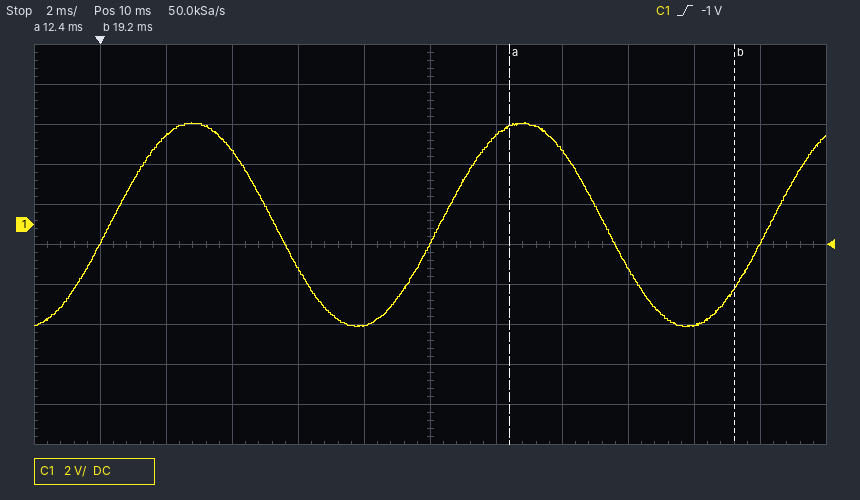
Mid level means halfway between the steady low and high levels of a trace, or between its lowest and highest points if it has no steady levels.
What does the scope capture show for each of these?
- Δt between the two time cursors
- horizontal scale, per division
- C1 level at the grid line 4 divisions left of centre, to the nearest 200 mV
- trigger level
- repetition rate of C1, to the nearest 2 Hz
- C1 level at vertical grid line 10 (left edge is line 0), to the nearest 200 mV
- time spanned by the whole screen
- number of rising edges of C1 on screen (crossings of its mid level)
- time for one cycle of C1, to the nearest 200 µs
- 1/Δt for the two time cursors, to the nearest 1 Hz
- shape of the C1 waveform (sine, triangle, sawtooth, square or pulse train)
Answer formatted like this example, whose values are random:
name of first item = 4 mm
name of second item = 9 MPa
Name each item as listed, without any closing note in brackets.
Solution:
Δt between the two time cursors = 6.8 ms
horizontal scale, per division = 2 ms
C1 level at the grid line 4 divisions left of centre, to the nearest 200 mV = 4.4 V
trigger level = -1 V
repetition rate of C1, to the nearest 2 Hz = 100 Hz
C1 level at vertical grid line 10 (left edge is line 0), to the nearest 200 mV = -5.0 V
time spanned by the whole screen = 24 ms
number of rising edges of C1 on screen = 3
time for one cycle of C1, to the nearest 200 µs = 10.0 ms
1/Δt for the two time cursors, to the nearest 1 Hz = 147 Hz
shape of the C1 waveform = sine
